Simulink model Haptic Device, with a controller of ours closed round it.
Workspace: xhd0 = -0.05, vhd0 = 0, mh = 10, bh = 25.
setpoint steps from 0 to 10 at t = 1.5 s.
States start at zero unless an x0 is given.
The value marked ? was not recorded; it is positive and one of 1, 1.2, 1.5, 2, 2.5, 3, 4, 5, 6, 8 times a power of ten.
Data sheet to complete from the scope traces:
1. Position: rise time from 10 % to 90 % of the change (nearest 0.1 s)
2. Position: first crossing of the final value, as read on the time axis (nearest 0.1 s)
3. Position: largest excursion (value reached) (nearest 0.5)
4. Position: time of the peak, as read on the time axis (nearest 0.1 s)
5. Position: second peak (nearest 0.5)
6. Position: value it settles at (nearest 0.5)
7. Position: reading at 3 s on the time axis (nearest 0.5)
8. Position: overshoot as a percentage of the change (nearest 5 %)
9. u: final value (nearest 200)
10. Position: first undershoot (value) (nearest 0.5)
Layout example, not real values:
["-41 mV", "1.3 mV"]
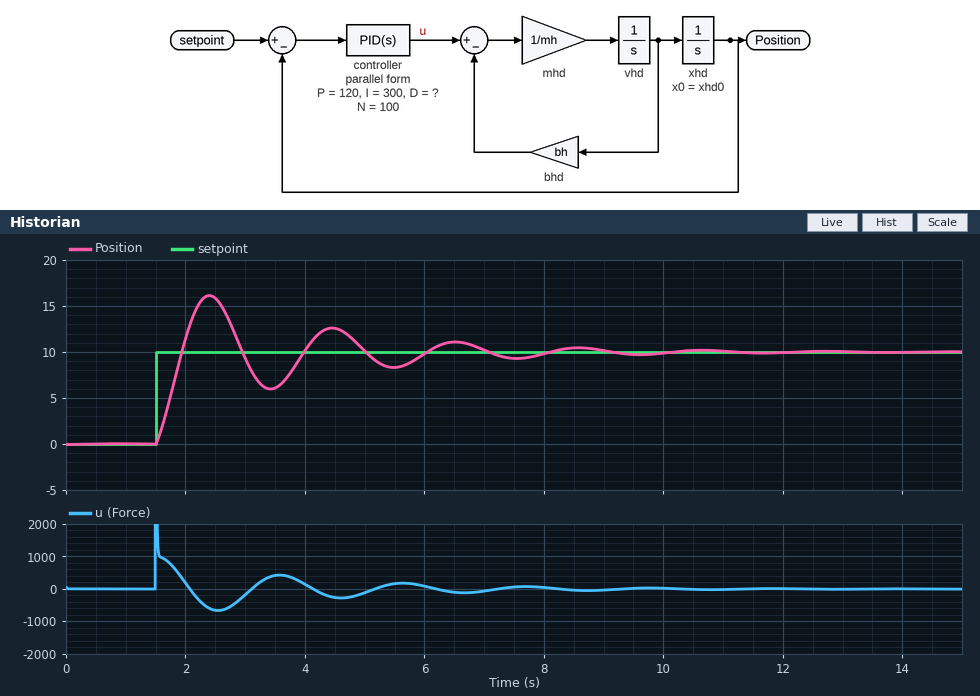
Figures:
["0.3 s", "1.9 s", "16.0", "2.4 s", "12.5", "10.0", "9.5", "60 %", "0", "6.0"]
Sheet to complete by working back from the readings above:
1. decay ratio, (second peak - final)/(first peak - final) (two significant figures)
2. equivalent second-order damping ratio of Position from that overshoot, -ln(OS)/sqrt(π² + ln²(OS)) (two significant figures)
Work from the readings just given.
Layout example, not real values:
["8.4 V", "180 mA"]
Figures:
["0.42", "0.16"]
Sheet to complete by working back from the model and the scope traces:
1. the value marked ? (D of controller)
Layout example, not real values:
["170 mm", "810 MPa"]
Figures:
["15"]
